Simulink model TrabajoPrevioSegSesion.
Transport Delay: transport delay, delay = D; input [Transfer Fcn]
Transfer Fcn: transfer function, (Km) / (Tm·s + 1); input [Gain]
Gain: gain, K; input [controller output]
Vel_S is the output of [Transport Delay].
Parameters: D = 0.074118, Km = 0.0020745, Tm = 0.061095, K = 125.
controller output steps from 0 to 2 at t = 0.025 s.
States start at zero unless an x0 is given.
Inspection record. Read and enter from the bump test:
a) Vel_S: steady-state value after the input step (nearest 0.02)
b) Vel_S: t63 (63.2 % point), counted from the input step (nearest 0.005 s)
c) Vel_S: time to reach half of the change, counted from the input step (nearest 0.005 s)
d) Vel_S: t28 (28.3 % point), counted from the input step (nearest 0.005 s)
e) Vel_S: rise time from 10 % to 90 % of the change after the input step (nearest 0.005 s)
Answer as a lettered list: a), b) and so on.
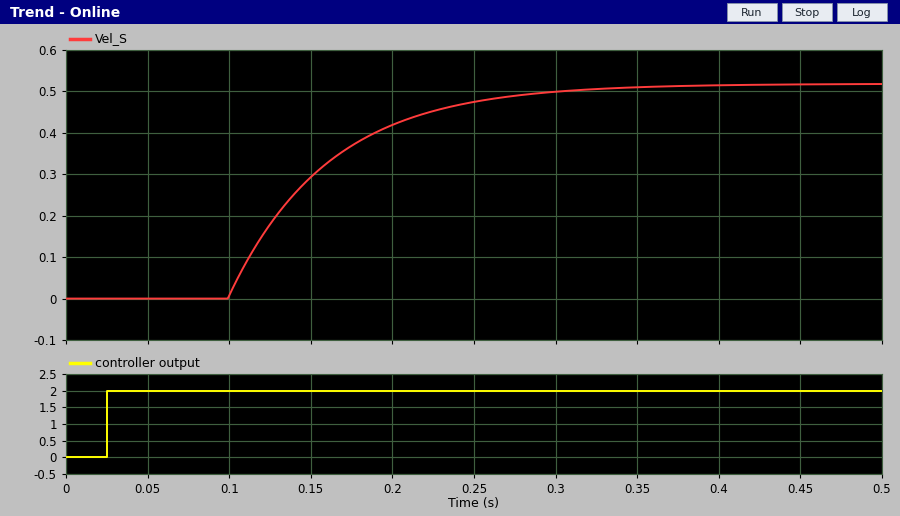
a) 0.52
b) 0.135 s
c) 0.115 s
d) 0.095 s
e) 0.135 s
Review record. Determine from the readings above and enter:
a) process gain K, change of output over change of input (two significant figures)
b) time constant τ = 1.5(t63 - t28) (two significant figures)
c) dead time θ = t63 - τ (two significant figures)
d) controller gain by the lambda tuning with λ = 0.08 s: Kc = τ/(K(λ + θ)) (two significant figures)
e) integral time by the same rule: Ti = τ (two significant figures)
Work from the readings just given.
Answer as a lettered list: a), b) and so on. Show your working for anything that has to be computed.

a) (0.52 - 0) / 2 = 0.26
b) 1.5 × (0.135 - 0.095) = 0.060 s
c) 0.135 - 0.06 = 0.075 s
d) 0.06 / (0.26 × (0.08 + 0.075)) = 1.5
e) 0.060 s
